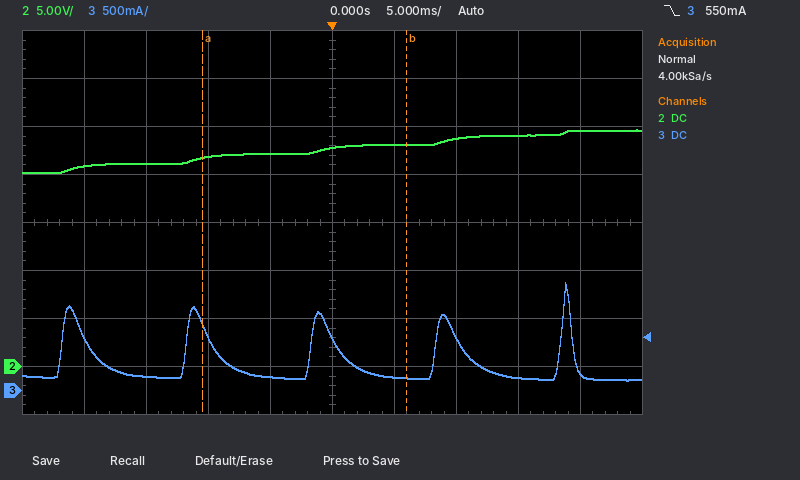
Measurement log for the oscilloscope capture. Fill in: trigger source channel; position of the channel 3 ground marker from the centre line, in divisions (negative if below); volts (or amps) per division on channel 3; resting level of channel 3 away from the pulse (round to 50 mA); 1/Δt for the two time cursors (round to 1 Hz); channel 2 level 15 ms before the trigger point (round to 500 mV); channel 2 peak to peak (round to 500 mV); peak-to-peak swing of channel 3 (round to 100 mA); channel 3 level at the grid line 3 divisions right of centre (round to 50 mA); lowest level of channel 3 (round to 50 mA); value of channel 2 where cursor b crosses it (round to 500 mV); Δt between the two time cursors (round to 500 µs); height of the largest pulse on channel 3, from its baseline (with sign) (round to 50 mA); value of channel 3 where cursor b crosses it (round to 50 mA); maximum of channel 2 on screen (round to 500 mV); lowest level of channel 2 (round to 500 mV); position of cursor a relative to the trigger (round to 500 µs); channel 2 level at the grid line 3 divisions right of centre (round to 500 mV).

channel 3
-3.5 div
500 mA
150 mA
61 Hz
21.0 V
4.5 V
1.00 A
150 mA
100 mA
23.0 V
16.5 ms
+1.00 A
150 mA
24.5 V
20.0 V
-10.5 ms
24.0 V
